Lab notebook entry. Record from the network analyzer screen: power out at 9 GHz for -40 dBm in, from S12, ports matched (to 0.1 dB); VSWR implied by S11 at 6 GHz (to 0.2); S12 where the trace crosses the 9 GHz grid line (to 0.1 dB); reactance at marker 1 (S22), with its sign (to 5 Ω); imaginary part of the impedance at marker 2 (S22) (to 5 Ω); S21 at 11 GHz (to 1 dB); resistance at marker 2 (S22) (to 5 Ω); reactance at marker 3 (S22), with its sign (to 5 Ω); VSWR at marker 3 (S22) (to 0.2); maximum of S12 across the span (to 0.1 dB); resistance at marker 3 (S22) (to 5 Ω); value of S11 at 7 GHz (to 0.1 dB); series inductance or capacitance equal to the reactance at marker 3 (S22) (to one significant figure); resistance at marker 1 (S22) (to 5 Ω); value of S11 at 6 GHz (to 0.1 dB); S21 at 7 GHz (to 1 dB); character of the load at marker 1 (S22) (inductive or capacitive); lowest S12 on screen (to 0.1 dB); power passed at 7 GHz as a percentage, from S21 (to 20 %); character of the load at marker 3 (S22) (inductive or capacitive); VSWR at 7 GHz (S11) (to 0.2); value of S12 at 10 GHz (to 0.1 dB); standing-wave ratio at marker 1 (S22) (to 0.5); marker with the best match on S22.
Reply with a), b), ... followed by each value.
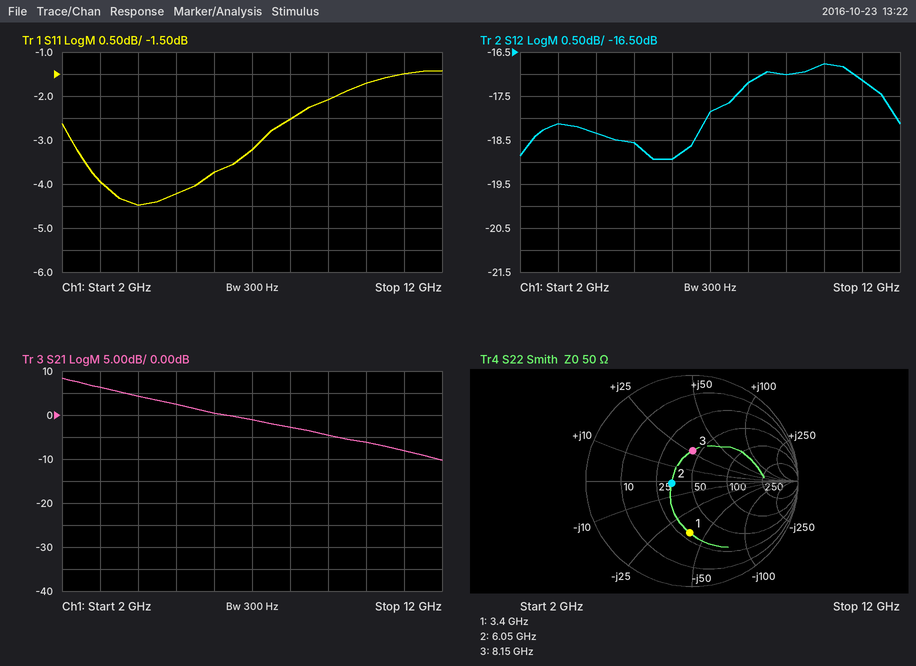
a) -57.0 dBm
b) 4.8
c) -17.0 dB
d) -40 Ω
e) 0 Ω
f) -8 dB
g) 35 Ω
h) +25 Ω
i) 1.8
j) -16.8 dB
k) 45 Ω
l) -3.2 dB
m) 500 pH
n) 30 Ω
o) -3.7 dB
p) -1 dB
q) capacitive
r) -18.9 dB
s) 80 %
t) inductive
u) 5.4
v) -16.8 dB
w) 3.0
x) marker 2
